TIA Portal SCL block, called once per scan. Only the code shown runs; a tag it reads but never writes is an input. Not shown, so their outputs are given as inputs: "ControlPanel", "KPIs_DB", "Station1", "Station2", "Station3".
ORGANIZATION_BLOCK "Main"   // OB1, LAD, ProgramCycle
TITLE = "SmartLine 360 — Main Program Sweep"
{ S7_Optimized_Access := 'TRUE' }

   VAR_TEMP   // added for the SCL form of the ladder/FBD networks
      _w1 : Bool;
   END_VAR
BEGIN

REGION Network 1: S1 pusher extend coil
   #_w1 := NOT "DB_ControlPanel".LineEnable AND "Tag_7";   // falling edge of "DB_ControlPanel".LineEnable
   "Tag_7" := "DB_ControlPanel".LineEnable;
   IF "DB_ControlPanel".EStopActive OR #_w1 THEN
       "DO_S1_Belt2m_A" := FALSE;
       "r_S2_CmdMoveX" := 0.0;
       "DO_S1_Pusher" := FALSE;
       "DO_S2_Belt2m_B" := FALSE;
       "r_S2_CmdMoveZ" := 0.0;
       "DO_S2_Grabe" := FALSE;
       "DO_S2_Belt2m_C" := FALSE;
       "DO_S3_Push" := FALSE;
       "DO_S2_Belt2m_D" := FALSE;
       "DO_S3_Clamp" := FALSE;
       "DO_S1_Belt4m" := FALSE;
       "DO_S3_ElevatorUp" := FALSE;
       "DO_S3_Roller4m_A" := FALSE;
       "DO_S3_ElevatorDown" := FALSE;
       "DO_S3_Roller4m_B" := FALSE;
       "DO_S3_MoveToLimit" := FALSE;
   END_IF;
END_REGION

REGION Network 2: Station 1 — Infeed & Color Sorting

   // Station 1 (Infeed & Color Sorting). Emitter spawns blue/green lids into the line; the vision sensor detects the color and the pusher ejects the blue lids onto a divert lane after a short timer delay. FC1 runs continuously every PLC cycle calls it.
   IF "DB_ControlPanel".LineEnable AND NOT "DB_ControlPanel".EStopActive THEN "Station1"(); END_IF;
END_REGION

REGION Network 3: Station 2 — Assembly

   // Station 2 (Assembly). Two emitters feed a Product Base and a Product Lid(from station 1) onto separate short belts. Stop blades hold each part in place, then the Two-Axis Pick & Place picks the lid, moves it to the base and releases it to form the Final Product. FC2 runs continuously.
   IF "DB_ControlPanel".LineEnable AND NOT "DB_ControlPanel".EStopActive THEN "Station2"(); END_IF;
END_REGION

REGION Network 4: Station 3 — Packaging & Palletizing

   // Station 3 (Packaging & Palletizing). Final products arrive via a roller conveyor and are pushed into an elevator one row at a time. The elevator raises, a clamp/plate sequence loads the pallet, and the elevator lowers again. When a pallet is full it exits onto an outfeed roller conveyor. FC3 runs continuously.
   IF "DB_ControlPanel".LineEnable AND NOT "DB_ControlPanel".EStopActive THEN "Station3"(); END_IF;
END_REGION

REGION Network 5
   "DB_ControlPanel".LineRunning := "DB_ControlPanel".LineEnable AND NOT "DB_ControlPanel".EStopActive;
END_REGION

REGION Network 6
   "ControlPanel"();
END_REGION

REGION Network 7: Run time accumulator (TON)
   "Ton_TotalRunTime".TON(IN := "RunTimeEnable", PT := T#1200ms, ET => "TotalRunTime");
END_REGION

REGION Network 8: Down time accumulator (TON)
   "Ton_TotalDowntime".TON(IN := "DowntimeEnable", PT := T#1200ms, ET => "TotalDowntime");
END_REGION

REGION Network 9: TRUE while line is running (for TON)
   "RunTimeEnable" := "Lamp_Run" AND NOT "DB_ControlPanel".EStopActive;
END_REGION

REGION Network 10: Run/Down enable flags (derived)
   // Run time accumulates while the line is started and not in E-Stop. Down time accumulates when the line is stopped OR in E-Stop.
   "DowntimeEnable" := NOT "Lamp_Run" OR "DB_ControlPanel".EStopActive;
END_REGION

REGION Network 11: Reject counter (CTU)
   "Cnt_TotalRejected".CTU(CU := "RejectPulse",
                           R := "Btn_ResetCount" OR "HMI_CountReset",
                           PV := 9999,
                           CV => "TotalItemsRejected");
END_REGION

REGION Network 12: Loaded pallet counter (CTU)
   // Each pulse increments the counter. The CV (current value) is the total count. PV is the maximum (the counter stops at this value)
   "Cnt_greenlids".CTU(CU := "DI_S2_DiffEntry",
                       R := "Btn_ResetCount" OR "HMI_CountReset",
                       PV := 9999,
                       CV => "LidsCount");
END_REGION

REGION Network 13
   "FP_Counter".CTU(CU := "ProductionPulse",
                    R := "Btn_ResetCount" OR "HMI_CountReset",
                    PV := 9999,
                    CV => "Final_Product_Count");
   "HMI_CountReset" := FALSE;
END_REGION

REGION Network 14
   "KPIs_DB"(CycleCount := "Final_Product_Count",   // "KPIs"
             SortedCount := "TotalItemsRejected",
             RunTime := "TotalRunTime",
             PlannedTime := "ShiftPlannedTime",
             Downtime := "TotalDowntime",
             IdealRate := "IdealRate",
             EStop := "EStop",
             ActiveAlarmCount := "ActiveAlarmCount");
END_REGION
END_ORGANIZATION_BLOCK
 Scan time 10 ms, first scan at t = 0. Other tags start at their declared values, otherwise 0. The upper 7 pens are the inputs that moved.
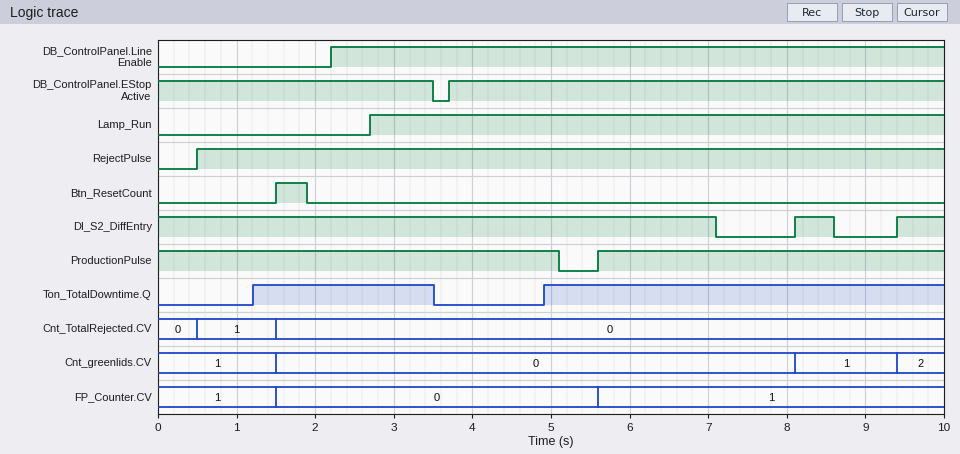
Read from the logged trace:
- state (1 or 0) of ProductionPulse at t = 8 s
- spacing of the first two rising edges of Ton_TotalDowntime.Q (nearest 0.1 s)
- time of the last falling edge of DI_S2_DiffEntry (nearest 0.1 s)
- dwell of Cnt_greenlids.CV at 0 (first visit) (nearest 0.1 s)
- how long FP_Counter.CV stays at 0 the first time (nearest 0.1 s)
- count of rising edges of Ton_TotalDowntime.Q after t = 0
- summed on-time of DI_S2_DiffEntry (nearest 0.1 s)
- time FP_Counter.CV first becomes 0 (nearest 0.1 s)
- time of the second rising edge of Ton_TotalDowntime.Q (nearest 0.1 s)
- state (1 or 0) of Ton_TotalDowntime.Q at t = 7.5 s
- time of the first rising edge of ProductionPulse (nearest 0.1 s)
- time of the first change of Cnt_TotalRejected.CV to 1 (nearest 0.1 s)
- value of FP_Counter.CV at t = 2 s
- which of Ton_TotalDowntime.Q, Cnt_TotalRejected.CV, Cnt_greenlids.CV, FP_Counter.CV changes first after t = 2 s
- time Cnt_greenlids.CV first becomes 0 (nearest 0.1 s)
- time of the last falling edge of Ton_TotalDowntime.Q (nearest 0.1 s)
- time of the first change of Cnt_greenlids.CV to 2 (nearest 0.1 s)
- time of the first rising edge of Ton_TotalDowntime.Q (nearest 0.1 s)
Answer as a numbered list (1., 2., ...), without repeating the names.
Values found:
1. 1
2. 3.7 s
3. 8.6 s
4. 6.6 s
5. 4.1 s
6. 2
7. 8.2 s
8. 1.5 s
9. 4.9 s
10. 1
11. 5.6 s
12. 0.5 s
13. 0
14. Ton_TotalDowntime.Q
15. 1.5 s
16. 3.5 s
17. 9.4 s
18. 1.2 s
